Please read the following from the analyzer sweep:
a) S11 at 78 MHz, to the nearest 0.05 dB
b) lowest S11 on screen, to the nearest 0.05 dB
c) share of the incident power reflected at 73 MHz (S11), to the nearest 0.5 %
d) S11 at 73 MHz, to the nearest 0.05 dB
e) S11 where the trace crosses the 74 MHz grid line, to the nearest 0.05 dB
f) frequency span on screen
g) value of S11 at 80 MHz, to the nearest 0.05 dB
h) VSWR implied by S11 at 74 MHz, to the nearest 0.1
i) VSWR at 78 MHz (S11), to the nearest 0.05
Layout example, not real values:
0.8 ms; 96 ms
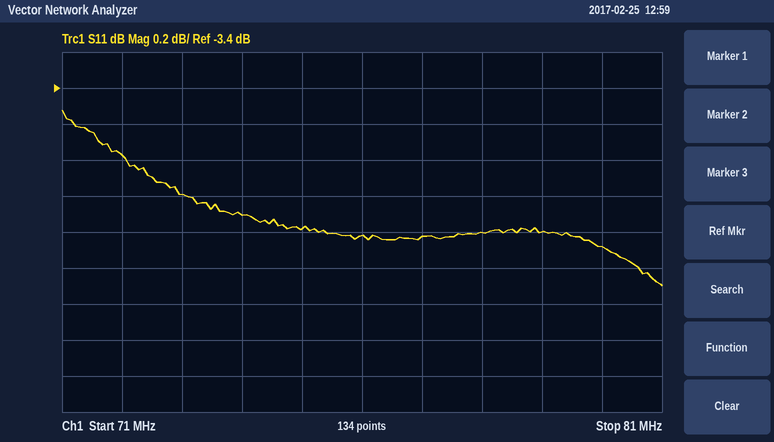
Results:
-4.20 dB; -4.50 dB; 40.0 %; -4.00 dB; -4.10 dB; 10 MHz; -4.30 dB; 4.3; 4.20
